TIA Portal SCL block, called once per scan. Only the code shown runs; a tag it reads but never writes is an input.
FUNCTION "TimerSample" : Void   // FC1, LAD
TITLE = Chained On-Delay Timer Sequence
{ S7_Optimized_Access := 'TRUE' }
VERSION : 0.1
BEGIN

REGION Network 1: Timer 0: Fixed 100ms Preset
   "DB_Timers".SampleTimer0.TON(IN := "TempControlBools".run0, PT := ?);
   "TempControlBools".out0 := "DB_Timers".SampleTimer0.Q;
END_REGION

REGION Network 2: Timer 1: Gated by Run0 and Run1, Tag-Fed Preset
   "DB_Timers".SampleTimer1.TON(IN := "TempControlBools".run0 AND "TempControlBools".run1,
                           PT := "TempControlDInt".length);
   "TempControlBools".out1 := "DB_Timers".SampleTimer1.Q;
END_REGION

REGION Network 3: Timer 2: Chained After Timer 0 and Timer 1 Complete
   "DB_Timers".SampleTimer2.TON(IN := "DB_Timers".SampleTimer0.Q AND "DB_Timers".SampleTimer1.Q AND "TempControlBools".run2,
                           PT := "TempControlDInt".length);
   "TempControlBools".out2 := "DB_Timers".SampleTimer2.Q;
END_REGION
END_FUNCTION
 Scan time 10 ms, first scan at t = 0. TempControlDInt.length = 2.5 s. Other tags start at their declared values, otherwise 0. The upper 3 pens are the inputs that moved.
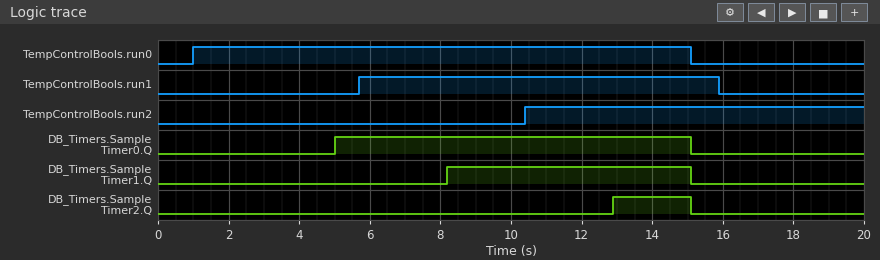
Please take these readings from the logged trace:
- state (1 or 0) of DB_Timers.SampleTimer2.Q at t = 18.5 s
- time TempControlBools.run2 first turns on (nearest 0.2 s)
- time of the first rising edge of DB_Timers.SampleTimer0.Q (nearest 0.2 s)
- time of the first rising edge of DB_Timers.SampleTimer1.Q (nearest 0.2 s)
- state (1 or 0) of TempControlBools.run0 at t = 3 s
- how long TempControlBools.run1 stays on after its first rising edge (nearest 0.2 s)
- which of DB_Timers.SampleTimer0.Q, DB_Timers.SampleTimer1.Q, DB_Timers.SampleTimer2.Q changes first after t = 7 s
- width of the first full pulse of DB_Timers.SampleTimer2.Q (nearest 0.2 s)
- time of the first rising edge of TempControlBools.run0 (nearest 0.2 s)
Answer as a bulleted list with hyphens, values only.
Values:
- 0
- 10.4 s
- 5.0 s
- 8.2 s
- 1
- 10.2 s
- DB_Timers.SampleTimer1.Q
- 2.2 s
- 1.0 s
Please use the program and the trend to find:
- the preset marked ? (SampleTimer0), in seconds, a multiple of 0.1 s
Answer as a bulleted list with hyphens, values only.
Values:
- 4.0 s
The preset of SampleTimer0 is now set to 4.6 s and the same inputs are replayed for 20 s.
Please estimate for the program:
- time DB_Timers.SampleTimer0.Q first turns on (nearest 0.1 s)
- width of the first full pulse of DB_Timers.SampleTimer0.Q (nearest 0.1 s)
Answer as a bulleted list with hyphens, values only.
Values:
- 5.6 s
- 9.5 s
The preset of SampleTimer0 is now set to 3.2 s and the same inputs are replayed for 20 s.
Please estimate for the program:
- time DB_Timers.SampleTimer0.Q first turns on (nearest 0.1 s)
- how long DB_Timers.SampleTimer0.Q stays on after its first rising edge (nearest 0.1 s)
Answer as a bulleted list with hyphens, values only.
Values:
- 4.2 s
- 10.9 s
